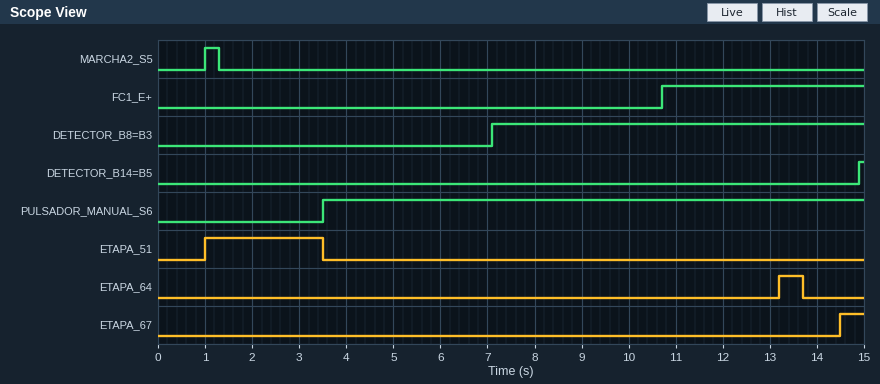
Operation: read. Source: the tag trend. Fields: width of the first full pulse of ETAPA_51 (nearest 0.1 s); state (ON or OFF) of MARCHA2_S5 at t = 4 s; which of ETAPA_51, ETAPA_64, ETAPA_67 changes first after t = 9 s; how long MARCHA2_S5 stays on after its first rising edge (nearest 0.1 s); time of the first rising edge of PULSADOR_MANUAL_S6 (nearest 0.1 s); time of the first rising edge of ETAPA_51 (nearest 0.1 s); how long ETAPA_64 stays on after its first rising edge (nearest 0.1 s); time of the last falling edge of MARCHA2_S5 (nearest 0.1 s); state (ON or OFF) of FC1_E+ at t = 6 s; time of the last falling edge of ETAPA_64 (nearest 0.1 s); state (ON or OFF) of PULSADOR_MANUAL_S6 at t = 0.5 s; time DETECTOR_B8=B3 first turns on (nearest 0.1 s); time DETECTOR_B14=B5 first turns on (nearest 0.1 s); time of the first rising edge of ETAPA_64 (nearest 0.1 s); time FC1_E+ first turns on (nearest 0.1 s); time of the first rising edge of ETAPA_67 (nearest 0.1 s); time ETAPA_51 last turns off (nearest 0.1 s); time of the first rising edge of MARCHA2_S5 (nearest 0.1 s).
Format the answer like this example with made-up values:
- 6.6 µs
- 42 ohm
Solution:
- 2.5 s
- OFF
- ETAPA_64
- 0.3 s
- 3.5 s
- 1.0 s
- 0.5 s
- 1.3 s
- OFF
- 13.7 s
- OFF
- 7.1 s
- 14.9 s
- 13.2 s
- 10.7 s
- 14.5 s
- 3.5 s
- 1.0 s
